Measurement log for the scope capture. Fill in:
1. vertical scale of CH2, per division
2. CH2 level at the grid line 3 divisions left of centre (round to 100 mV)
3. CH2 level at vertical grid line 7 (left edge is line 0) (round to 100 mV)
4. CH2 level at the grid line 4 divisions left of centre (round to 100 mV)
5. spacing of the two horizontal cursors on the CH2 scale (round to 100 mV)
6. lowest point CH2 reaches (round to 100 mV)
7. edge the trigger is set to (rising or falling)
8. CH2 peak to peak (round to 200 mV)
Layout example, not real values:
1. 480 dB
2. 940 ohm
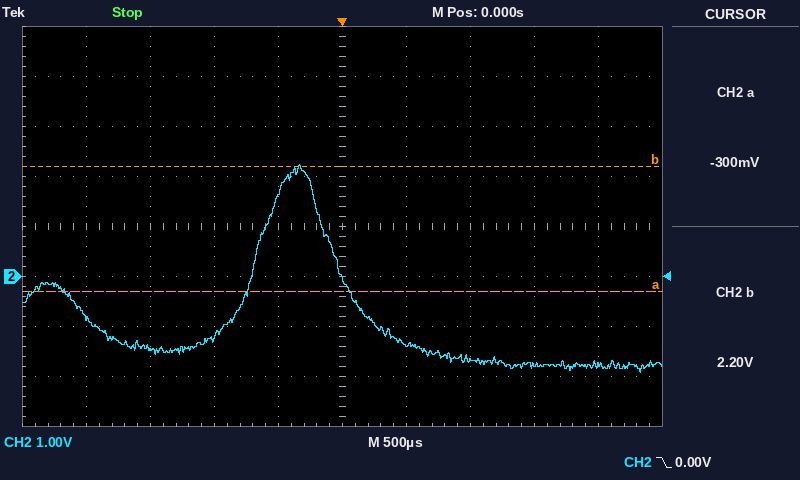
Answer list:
1. 1 V
2. -1.4 V
3. -1.7 V
4. -800 mV
5. 2.5 V
6. -1.9 V
7. falling
8. 4.2 V
